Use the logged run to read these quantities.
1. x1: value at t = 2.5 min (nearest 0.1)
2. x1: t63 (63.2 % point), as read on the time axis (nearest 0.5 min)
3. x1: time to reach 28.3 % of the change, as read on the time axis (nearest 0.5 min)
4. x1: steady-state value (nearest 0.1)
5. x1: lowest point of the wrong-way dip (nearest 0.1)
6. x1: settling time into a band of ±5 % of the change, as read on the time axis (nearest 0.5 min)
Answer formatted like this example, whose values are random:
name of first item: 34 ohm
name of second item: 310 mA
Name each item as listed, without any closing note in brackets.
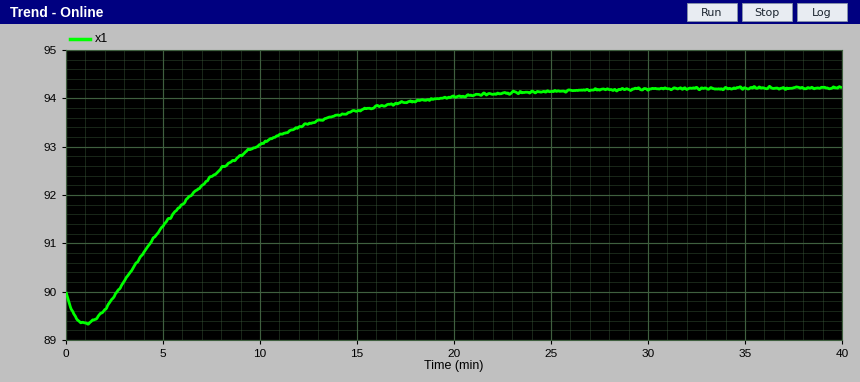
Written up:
x1: value at t = 2.5 min: 89.9
x1: t63 (63.2 % point), as read on the time axis: 8.5 min
x1: time to reach 28.3 % of the change, as read on the time axis: 4.5 min
x1: steady-state value: 94.2
x1: lowest point of the wrong-way dip: 89.3
x1: settling time into a band of ±5 % of the change, as read on the time axis: 19.5 min
